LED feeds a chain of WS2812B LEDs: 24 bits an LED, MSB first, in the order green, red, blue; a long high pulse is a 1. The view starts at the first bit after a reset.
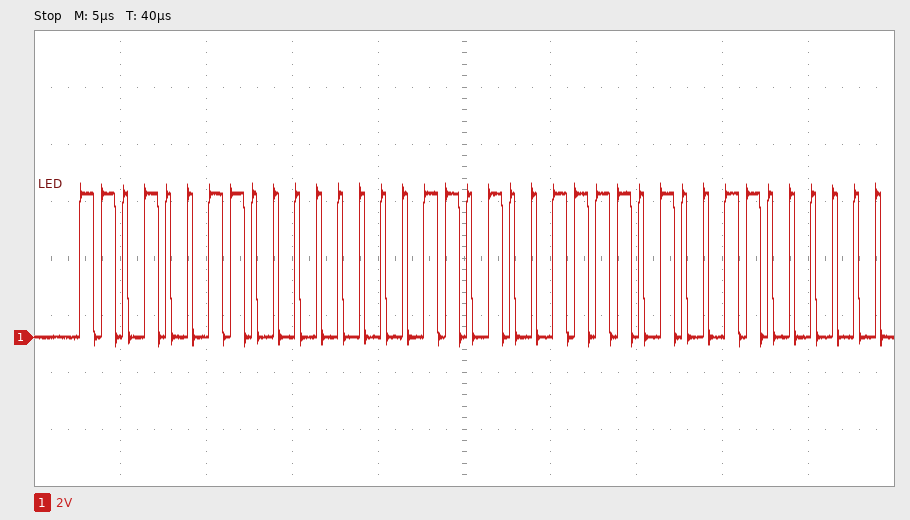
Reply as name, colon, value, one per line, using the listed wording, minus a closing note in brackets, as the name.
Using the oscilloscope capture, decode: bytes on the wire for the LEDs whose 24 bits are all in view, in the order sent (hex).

bytes on the wire for the LEDs whose 24 bits are all in view, in the order sent: D3 00 D3
